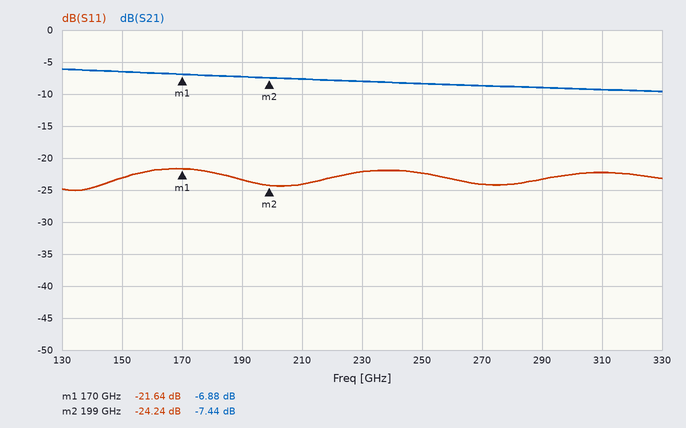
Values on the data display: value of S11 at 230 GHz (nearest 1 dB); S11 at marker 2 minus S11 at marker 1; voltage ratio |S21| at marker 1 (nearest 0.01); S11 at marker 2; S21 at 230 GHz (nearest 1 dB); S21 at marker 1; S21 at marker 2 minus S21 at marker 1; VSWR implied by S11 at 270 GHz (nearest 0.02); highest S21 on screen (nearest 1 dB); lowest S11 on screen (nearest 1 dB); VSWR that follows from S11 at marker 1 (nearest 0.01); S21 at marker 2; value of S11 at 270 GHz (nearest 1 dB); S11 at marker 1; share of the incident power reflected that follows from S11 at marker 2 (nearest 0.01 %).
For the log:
-22 dB
-2.60 dB
0.45
-24.24 dB
-8 dB
-6.88 dB
-0.56 dB
1.14
-6 dB
-25 dB
1.18
-7.44 dB
-24 dB
-21.64 dB
0.38 %
